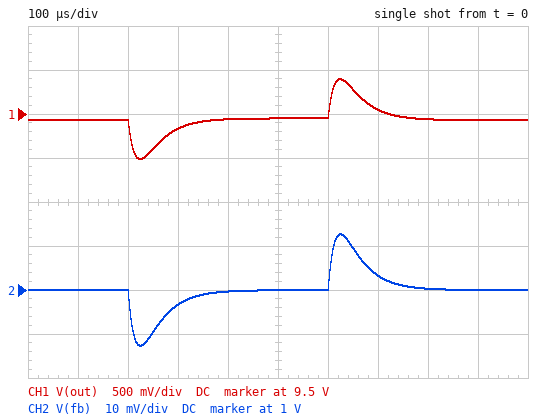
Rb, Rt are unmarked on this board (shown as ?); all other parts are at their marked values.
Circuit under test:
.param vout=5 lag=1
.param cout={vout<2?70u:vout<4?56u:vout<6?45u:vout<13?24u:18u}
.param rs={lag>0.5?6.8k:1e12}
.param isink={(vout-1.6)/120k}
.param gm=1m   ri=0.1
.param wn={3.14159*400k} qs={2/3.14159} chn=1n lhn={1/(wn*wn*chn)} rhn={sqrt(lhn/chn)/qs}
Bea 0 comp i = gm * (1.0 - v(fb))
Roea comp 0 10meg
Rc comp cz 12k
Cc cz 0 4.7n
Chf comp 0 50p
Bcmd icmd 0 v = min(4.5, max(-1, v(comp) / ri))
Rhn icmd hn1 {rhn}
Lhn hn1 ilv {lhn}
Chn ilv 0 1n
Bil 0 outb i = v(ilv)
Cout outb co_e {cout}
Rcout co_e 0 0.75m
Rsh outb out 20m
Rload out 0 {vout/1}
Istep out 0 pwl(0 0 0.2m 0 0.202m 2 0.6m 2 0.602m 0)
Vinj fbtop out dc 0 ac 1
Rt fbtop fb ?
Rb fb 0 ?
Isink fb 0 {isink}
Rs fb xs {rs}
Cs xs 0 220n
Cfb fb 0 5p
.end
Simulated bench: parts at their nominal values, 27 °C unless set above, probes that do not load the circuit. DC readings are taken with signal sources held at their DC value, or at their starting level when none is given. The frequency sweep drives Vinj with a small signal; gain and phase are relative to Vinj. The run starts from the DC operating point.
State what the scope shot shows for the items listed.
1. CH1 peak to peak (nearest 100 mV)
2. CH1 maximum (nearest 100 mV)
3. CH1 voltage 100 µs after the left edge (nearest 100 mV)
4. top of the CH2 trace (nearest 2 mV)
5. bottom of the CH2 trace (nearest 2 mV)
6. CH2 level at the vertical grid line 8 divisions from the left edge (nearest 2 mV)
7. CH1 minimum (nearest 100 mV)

900 mV
9.9 V
9.4 V
1.012 V
988 mV
1.000 V
9.0 V
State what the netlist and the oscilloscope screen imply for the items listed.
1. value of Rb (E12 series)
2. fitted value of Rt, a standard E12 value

100 kΩ
220 kΩ
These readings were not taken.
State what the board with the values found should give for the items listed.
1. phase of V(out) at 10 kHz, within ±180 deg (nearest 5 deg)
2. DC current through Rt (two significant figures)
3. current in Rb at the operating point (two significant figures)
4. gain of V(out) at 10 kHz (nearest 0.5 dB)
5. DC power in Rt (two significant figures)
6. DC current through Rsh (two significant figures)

135 deg
38 µA
10 µA
-0.5 dB
320 µW
1.9 A
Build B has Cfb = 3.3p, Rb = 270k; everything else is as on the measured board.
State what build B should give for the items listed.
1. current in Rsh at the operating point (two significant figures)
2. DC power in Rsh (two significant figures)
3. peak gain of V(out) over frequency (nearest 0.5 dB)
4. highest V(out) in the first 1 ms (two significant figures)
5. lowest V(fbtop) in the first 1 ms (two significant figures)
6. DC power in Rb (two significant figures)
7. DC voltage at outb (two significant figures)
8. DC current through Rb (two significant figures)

1.6 A
52 mW
1.0 dB
8.5 V
7.6 V
3.7 µW
8.1 V
3.7 µA
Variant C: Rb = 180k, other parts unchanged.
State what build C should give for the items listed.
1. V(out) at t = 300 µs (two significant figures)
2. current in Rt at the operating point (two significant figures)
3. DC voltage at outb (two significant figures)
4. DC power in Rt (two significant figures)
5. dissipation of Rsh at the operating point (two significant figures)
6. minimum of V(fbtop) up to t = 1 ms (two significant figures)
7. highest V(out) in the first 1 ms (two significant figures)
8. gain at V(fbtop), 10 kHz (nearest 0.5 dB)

8.4 V
34 µA
8.5 V
250 µW
57 mW
8.0 V
8.9 V
-2.5 dB
